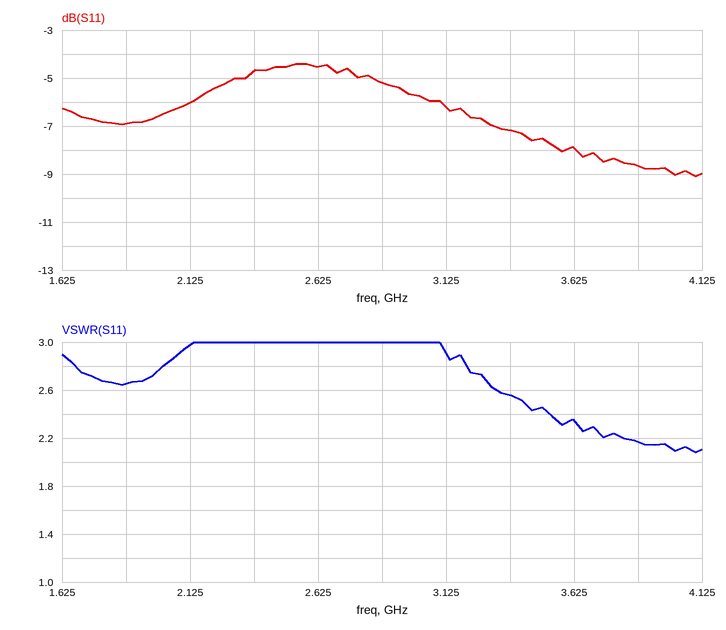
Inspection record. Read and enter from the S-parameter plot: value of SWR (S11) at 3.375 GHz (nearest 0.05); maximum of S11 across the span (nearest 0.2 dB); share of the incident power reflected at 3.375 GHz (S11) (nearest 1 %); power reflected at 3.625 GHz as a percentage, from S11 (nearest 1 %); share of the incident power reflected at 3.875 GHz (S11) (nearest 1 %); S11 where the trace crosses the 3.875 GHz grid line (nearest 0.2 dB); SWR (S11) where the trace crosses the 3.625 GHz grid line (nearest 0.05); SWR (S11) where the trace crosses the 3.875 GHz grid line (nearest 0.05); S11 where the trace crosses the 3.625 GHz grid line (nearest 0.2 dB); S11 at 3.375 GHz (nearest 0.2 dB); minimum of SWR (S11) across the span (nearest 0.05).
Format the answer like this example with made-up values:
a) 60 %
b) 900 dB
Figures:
a) 2.55
b) -4.4 dB
c) 19 %
d) 16 %
e) 14 %
f) -8.6 dB
g) 2.35
h) 2.15
i) -8.0 dB
j) -7.2 dB
k) 2.10
